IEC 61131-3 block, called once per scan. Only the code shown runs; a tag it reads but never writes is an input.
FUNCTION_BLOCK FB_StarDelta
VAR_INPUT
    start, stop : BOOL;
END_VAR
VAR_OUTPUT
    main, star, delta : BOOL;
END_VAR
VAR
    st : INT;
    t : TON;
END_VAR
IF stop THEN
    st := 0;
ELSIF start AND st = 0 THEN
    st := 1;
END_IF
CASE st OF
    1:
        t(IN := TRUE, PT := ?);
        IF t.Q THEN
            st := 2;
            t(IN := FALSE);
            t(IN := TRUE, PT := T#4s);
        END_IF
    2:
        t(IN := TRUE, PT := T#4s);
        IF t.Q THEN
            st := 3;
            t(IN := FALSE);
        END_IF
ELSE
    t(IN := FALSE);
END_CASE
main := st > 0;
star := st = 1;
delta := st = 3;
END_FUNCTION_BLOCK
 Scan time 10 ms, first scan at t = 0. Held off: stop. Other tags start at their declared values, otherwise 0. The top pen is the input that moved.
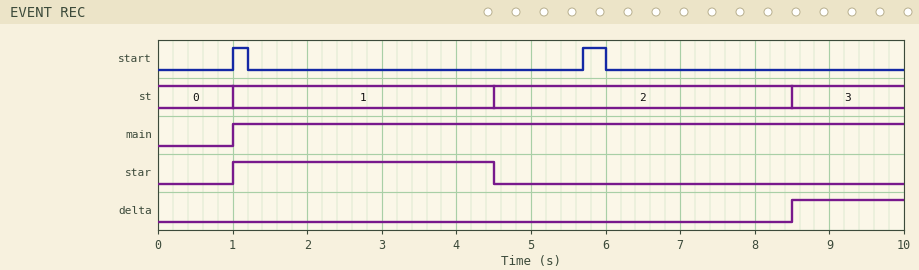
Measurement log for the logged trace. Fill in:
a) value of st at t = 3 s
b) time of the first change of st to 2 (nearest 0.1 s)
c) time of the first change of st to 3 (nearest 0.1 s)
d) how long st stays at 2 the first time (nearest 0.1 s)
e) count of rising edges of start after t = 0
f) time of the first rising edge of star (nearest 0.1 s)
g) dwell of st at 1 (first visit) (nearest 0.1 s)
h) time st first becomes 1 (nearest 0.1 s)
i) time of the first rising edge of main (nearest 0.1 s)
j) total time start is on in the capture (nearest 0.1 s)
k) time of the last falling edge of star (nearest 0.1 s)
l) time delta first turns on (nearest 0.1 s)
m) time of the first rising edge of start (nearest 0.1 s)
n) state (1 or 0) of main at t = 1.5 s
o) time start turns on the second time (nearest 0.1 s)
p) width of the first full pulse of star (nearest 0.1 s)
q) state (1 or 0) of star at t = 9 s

1
4.5 s
8.5 s
4.0 s
2
1.0 s
3.5 s
1.0 s
1.0 s
0.5 s
4.5 s
8.5 s
1.0 s
1
5.7 s
3.5 s
0
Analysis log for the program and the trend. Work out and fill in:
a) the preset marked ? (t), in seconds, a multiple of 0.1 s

3.5 s
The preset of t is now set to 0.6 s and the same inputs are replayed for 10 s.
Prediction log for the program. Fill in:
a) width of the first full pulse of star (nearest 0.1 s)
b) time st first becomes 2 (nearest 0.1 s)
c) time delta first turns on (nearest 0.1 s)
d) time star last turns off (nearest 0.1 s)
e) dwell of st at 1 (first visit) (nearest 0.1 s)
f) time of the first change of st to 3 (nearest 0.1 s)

0.6 s
1.6 s
5.6 s
1.6 s
0.6 s
5.6 s
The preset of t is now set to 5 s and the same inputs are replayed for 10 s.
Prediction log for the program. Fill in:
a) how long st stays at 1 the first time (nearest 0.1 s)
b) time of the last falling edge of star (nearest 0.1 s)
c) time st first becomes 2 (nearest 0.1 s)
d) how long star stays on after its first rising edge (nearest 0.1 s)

5.0 s
6.0 s
6.0 s
5.0 s
